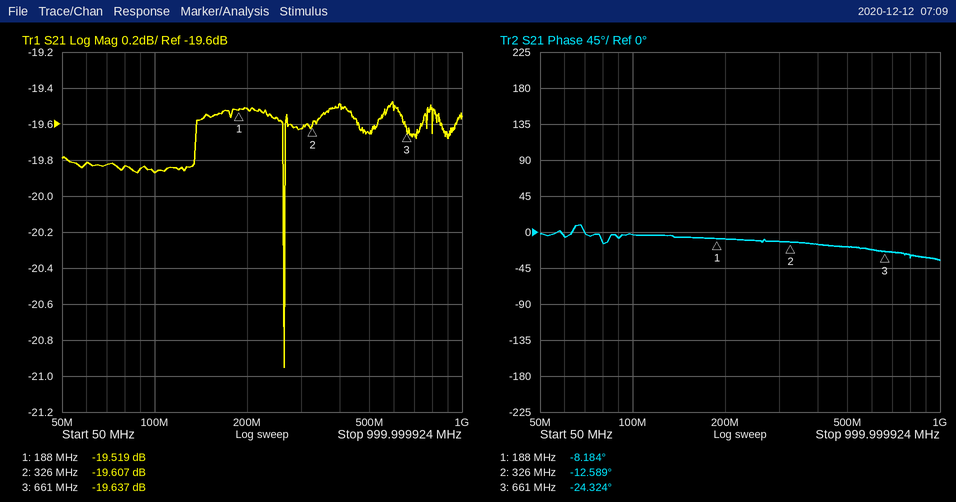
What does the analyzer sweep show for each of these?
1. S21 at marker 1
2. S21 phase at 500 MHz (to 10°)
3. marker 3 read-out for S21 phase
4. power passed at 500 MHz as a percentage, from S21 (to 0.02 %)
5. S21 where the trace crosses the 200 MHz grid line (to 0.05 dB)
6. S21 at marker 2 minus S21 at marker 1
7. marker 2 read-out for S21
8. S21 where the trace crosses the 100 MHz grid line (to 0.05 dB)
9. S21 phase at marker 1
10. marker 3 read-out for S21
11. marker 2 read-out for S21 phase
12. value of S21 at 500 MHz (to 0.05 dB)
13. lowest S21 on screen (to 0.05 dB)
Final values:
-19.519 dB
-20°
-24.324°
1.08 %
-19.50 dB
-0.088 dB
-19.607 dB
-19.85 dB
-8.184°
-19.637 dB
-12.589°
-19.65 dB
-20.95 dB
